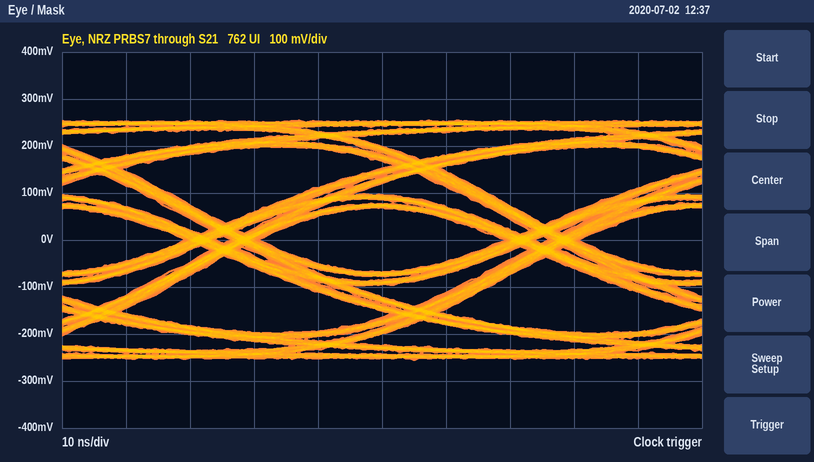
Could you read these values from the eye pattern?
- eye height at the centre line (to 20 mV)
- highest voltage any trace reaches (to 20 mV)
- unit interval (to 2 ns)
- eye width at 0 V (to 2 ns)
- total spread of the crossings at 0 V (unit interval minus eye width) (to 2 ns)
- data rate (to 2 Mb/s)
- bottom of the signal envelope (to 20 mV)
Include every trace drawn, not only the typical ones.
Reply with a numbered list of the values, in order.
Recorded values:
1. 140 mV
2. 260 mV
3. 50 ns
4. 38 ns
5. 12 ns
6. 20 Mb/s
7. -260 mV
